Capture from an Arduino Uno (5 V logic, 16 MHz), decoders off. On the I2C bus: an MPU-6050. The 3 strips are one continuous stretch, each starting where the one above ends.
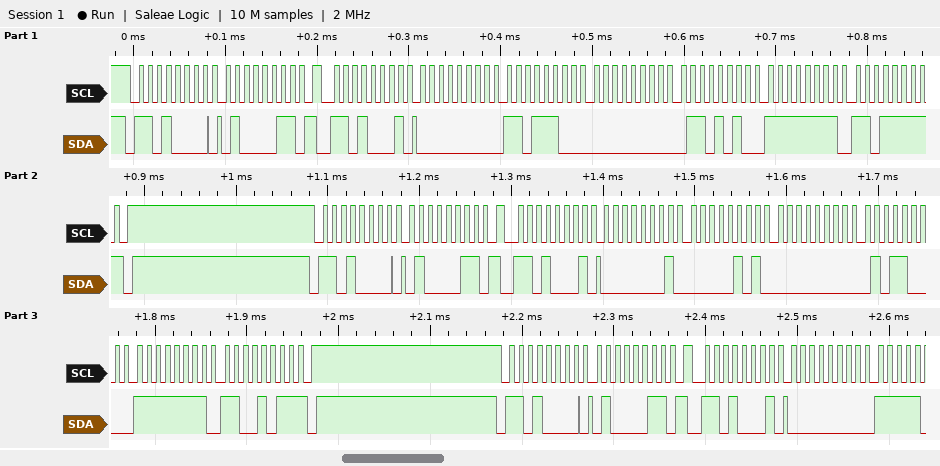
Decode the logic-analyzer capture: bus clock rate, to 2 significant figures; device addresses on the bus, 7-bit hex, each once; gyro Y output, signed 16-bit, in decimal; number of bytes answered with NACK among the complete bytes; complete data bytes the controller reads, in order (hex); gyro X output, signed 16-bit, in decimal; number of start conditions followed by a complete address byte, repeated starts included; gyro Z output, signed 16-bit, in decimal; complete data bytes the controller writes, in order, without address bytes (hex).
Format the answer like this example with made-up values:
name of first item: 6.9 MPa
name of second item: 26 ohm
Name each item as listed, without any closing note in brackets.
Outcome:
bus clock rate, to 2 significant figures: 100 kHz
device addresses on the bus, 7-bit hex, each once: 0x68
gyro Y output, signed 16-bit, in decimal: 106
number of bytes answered with NACK among the complete bytes: 2
complete data bytes the controller reads, in order: 00 DC 00 6A FF DF 01 05 00 58 FF CB 00
gyro X output, signed 16-bit, in decimal: 220
number of start conditions followed by a complete address byte, repeated starts included: 6
gyro Z output, signed 16-bit, in decimal: -33
complete data bytes the controller writes, in order, without address bytes: 43 43 43
